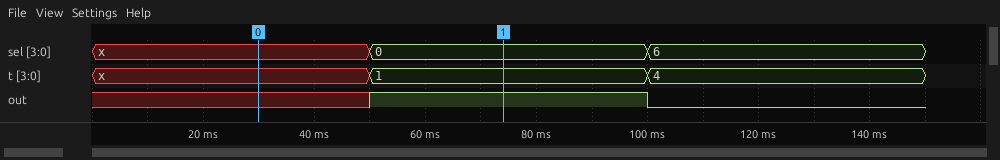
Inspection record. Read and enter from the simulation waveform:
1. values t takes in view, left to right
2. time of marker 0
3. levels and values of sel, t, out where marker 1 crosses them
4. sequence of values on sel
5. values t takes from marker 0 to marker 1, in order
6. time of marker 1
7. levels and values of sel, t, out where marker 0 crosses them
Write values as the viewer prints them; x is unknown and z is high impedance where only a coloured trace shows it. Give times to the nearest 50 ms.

x, 1, 4
50 ms
sel=0, t=1, out=1
x, 0, 6
x, 1
50 ms
sel=x, t=x, out=x
